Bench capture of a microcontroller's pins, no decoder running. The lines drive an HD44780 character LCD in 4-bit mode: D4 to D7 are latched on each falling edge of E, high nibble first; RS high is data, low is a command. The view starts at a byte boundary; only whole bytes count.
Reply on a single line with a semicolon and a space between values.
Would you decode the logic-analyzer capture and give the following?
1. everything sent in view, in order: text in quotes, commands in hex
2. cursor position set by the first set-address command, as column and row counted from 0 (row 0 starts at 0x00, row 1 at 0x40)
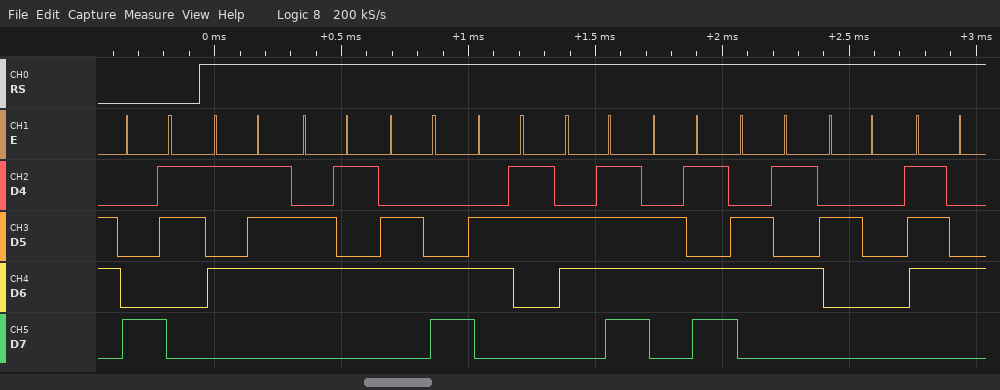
0x83 "Welcome t"; column 3, row 0
